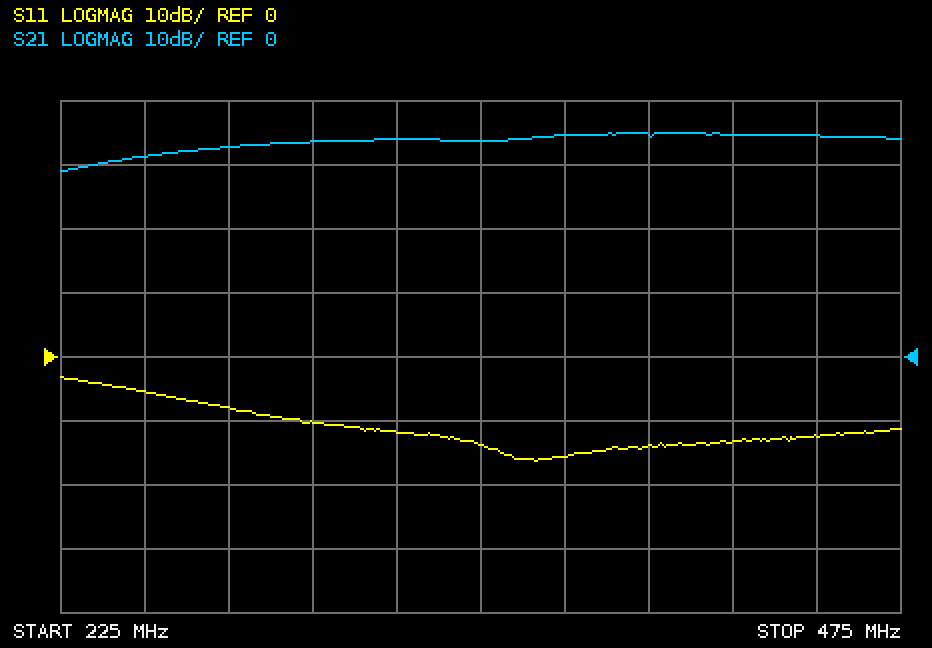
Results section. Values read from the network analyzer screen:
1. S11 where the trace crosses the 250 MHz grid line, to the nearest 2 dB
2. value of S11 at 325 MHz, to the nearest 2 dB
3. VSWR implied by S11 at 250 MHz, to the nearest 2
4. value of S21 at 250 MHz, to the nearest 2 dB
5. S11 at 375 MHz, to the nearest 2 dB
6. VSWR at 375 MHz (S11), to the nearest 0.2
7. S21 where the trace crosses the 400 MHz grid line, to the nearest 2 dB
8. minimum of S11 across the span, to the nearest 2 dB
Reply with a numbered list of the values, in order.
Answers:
1. -6 dB
2. -12 dB
3. 4
4. 32 dB
5. -16 dB
6. 1.4
7. 34 dB
8. -16 dB
